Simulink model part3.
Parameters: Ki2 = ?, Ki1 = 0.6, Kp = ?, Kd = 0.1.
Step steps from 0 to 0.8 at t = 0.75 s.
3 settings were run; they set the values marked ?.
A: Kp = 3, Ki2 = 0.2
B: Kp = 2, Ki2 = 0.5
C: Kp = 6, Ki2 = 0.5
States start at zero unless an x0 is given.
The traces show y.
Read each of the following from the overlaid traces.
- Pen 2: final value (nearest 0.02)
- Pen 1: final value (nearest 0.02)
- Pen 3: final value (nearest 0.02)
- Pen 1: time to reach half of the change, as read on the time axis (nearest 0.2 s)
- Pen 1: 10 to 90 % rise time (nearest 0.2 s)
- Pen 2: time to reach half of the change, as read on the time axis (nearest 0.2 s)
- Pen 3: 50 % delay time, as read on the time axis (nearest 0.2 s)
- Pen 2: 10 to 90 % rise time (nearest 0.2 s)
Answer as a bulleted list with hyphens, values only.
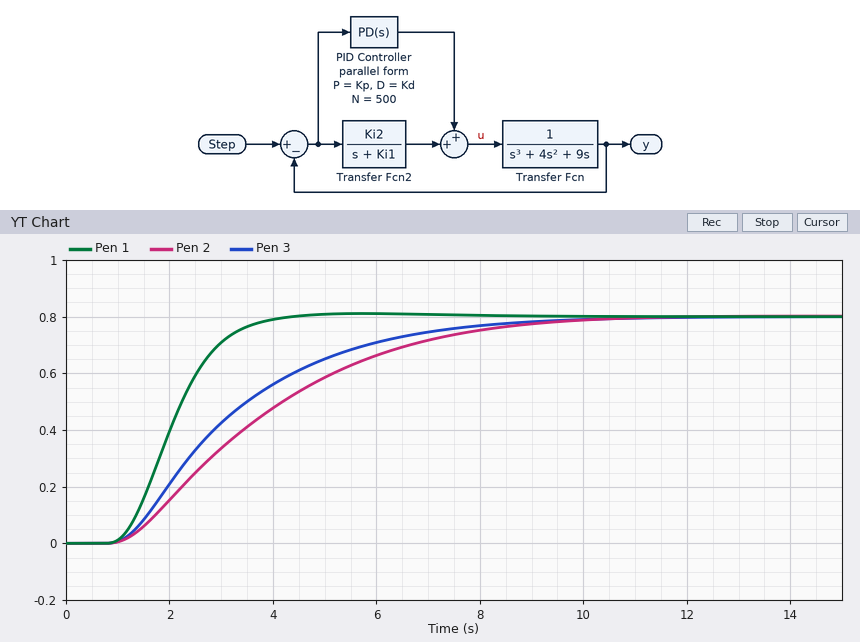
- 0.80
- 0.80
- 0.80
- 2.0 s
- 1.8 s
- 3.4 s
- 2.8 s
- 5.4 s
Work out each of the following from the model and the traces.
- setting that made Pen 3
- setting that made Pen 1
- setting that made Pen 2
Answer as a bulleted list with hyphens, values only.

- A
- C
- B
